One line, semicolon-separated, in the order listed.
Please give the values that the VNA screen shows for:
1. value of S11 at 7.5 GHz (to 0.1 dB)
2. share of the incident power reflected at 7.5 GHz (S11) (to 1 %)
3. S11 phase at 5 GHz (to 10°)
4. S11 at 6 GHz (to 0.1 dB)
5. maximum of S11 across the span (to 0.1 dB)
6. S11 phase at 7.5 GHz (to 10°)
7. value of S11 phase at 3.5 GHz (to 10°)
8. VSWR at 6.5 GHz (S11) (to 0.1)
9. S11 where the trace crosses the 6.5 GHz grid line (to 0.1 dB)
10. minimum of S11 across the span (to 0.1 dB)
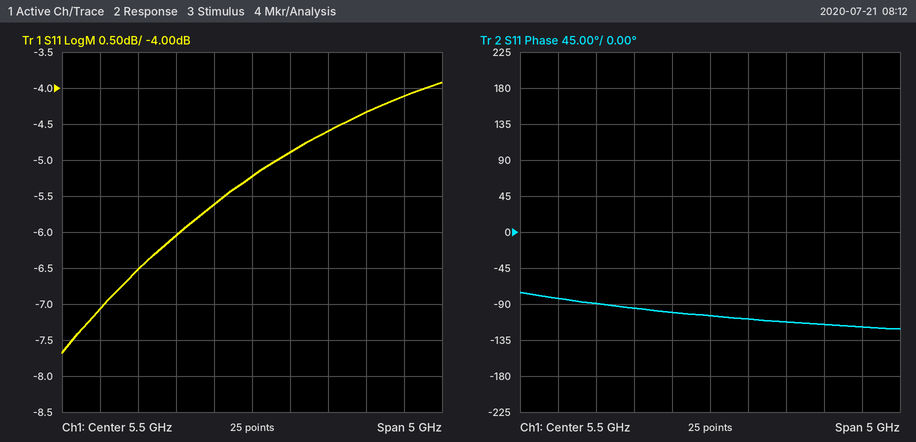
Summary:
-4.1 dB; 39 %; -100°; -4.9 dB; -3.9 dB; -120°; -80°; 3.9; -4.6 dB; -7.7 dB
